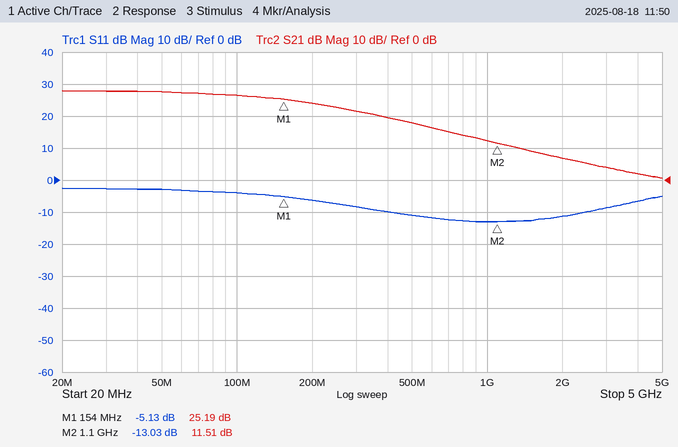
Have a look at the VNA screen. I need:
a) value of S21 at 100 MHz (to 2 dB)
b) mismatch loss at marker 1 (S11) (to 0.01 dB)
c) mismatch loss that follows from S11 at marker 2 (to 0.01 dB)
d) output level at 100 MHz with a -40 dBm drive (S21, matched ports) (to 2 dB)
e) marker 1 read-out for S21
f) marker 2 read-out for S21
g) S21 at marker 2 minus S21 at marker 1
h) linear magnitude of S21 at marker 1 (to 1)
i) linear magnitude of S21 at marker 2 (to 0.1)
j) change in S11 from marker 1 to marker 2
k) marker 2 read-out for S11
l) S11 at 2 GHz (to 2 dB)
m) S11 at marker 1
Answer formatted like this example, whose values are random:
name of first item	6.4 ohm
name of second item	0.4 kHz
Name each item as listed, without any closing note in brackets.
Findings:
value of S21 at 100 MHz	26 dB
mismatch loss at marker 1 (S11)	1.59 dB
mismatch loss that follows from S11 at marker 2	0.22 dB
output level at 100 MHz with a -40 dBm drive (S21, matched ports)	-14 dBm
marker 1 read-out for S21	25.19 dB
marker 2 read-out for S21	11.51 dB
S21 at marker 2 minus S21 at marker 1	-13.68 dB
linear magnitude of S21 at marker 1	18
linear magnitude of S21 at marker 2	3.8
change in S11 from marker 1 to marker 2	-7.90 dB
marker 2 read-out for S11	-13.03 dB
S11 at 2 GHz	-12 dB
S11 at marker 1	-5.13 dB
